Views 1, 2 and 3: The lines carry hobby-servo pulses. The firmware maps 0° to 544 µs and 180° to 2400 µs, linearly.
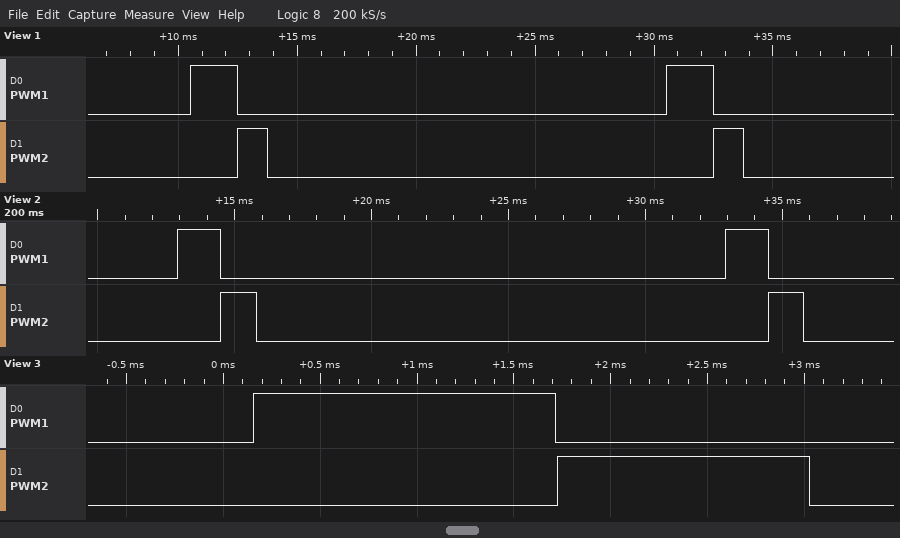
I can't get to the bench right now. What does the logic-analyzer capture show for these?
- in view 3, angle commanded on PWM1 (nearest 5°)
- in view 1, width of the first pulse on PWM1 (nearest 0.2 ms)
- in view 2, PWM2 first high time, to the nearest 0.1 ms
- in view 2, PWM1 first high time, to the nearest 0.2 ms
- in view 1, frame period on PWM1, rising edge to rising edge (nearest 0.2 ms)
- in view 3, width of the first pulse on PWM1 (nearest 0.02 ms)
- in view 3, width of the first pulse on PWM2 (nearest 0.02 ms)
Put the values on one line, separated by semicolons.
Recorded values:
100°; 2.0 ms; 1.3 ms; 1.6 ms; 20.0 ms; 1.56 ms; 1.30 ms
